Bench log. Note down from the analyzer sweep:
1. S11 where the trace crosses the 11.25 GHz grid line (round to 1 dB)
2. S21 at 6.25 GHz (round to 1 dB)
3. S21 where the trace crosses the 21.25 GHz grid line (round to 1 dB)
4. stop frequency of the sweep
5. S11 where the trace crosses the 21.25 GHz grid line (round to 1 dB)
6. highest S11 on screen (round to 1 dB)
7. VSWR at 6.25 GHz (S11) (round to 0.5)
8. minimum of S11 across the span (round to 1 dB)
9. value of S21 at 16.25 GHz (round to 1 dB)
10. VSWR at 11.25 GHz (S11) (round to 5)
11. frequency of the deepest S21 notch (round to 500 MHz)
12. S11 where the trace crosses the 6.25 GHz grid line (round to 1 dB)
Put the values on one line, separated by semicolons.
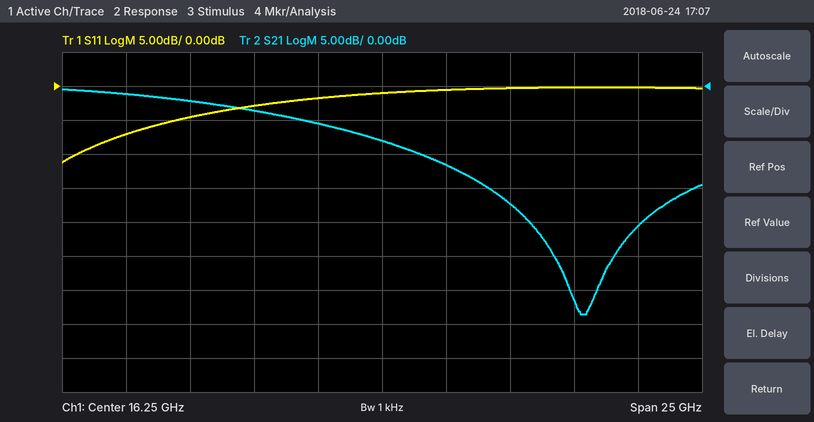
-3 dB; -1 dB; -17 dB; 28.75 GHz; 0 dB; 0 dB; 2.5; -11 dB; -8 dB; 5; 24.0 GHz; -7 dB
